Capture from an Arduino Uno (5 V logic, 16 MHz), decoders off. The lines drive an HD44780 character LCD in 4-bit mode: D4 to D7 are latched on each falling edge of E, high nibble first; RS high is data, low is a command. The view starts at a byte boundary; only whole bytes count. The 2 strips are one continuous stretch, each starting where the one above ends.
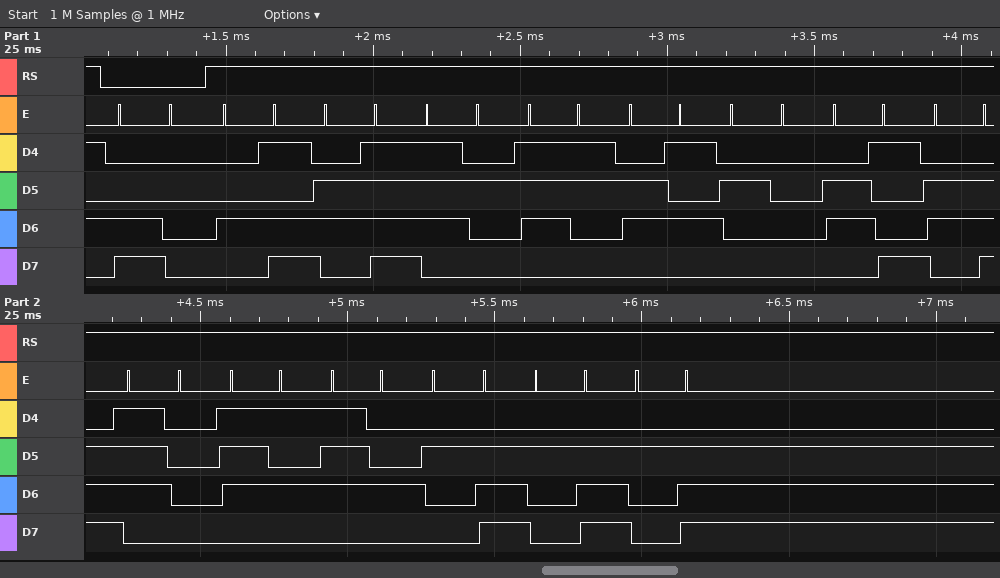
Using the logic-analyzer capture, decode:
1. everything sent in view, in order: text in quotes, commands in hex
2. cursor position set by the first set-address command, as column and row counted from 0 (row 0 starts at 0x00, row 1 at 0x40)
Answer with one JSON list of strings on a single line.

["0xC0 \"Morse input...\"", "column 0, row 1"]
